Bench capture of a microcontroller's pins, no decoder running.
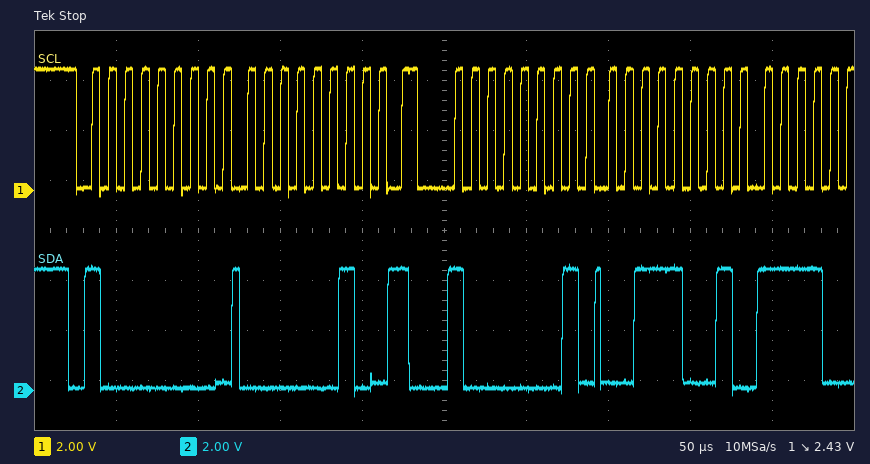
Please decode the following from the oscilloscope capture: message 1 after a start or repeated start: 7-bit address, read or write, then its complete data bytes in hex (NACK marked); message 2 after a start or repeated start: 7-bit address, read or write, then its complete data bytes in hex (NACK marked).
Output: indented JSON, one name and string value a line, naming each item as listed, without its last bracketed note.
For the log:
{
  "message 1 after a start or repeated start: 7-bit address, read or write, then its complete data bytes in hex": "0x40 write: 02",
  "message 2 after a start or repeated start: 7-bit address, read or write, then its complete data bytes in hex": "0x40 read: 39"
}
